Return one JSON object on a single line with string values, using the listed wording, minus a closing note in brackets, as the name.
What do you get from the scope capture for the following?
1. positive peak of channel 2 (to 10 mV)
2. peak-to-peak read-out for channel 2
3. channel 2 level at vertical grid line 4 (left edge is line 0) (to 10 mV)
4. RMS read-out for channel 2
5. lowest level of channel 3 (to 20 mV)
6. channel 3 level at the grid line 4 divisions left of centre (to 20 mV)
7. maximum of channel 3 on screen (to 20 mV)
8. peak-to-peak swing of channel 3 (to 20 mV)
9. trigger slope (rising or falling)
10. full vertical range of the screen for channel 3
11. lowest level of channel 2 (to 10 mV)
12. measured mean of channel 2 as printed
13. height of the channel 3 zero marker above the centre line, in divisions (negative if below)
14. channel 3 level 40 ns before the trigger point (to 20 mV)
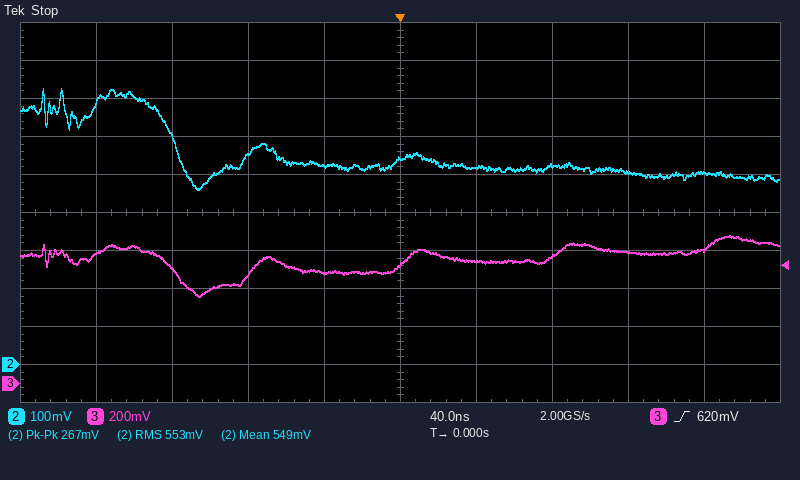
{"positive peak of channel 2": "730 mV", "peak-to-peak read-out for channel 2": "267 mV", "channel 2 level at vertical grid line 4 (left edge is line 0)": "520 mV", "RMS read-out for channel 2": "553 mV", "lowest level of channel 3": "460 mV", "channel 3 level at the grid line 4 divisions left of centre": "680 mV", "maximum of channel 3 on screen": "780 mV", "peak-to-peak swing of channel 3": "320 mV", "trigger slope": "rising", "full vertical range of the screen for channel 3": "2 V", "lowest level of channel 2": "460 mV", "measured mean of channel 2 as printed": "549 mV", "height of the channel 3 zero marker above the centre line, in divisions": "-4.5 div", "channel 3 level 40 ns before the trigger point": "580 mV"}
